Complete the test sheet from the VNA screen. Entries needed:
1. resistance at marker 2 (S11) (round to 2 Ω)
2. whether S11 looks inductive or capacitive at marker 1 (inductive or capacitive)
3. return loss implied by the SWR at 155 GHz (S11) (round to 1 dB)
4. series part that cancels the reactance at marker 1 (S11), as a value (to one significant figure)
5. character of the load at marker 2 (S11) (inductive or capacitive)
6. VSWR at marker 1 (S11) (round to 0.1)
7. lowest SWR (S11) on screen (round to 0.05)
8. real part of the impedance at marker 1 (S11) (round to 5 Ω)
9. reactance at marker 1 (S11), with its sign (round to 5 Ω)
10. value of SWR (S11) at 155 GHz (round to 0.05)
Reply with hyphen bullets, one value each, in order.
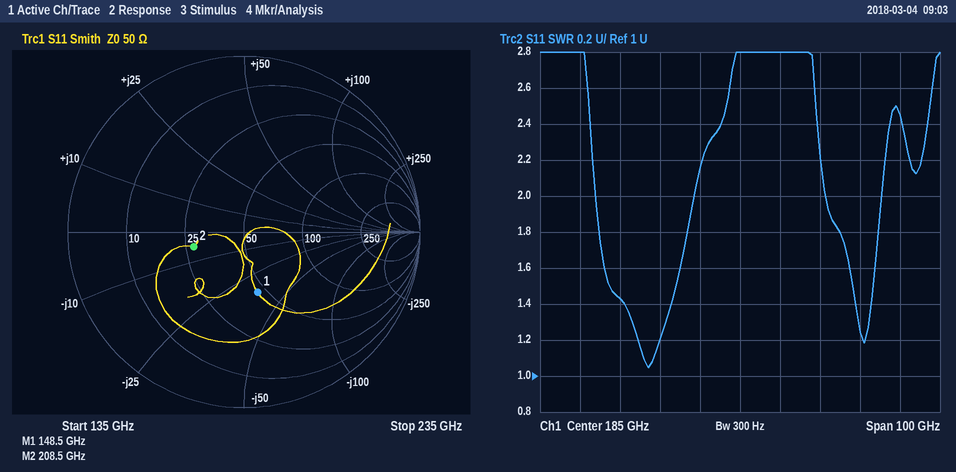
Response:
- 28 Ω
- capacitive
- 15 dB
- 40 pH
- capacitive
- 2.1
- 1.05
- 45 Ω
- -35 Ω
- 1.45
